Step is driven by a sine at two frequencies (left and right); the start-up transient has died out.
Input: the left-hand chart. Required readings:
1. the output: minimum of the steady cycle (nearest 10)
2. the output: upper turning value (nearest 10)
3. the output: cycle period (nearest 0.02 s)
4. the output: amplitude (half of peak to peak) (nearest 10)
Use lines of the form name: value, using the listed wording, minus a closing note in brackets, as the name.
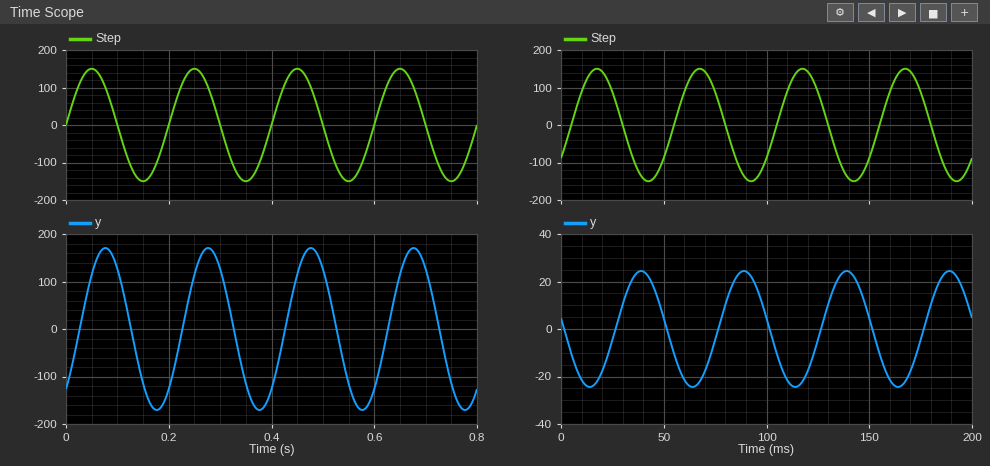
the output: minimum of the steady cycle: -170
the output: upper turning value: 170
the output: cycle period: 0.20 s
the output: amplitude (half of peak to peak): 170
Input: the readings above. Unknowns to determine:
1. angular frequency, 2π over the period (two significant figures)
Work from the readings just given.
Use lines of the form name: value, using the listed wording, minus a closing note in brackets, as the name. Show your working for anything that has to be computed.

angular frequency, 2π over the period: 2π / 0.2 = 31 rad/s
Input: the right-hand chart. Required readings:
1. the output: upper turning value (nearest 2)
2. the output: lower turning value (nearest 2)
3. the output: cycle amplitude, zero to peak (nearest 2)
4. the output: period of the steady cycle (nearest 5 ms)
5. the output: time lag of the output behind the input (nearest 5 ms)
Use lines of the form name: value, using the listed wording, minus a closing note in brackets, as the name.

the output: upper turning value: 24
the output: lower turning value: -24
the output: cycle amplitude, zero to peak: 24
the output: period of the steady cycle: 50 ms
the output: time lag of the output behind the input: 20 ms
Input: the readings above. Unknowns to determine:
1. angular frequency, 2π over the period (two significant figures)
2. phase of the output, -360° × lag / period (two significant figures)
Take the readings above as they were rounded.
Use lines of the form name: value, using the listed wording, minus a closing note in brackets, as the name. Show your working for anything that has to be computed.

angular frequency, 2π over the period: 2π / 50 = 0.13 rad/ms
phase of the output, -360° × lag / period: -360 × 20 / 50 = -140°
